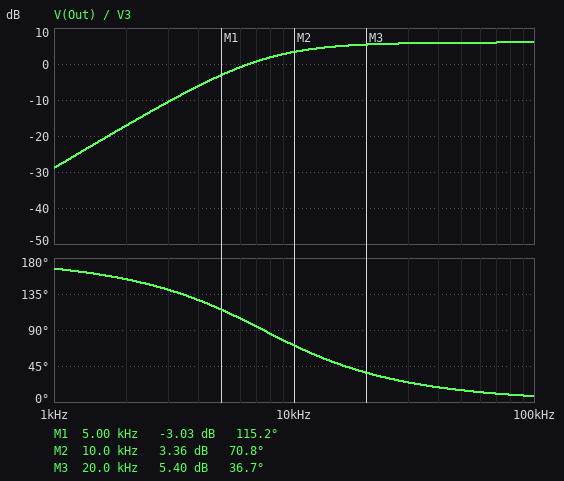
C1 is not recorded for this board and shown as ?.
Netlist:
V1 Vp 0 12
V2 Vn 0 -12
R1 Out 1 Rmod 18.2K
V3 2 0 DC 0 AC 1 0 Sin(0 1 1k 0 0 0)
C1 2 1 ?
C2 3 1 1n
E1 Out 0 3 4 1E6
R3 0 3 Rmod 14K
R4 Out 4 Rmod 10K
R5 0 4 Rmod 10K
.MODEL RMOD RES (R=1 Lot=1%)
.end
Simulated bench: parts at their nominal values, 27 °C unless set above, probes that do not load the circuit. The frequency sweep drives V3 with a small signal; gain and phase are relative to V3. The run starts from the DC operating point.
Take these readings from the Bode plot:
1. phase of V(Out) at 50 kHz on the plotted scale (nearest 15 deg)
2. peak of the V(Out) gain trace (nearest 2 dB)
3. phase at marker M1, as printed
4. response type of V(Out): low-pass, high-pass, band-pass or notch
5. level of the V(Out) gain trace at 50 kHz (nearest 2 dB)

15 deg
6 dB
115.2 deg
high-pass
6 dB
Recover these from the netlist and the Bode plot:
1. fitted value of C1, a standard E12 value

1.8 nF
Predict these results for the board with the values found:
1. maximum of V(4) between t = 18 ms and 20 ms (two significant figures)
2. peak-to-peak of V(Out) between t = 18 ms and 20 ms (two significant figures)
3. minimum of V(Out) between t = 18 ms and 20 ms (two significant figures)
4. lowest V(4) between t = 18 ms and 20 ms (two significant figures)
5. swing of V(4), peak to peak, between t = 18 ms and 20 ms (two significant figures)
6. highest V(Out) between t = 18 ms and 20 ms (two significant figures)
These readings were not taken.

18 mV
72 mV
-36 mV
-18 mV
36 mV
36 mV
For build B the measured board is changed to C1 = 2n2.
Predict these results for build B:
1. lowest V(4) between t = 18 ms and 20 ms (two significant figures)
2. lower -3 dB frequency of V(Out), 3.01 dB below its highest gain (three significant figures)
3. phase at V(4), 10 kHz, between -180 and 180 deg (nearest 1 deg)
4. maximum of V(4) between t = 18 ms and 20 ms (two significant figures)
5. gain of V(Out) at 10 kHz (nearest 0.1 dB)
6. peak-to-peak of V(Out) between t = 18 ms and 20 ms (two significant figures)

-22 mV
9.49 kHz
66 deg
22 mV
3.3 dB
87 mV
